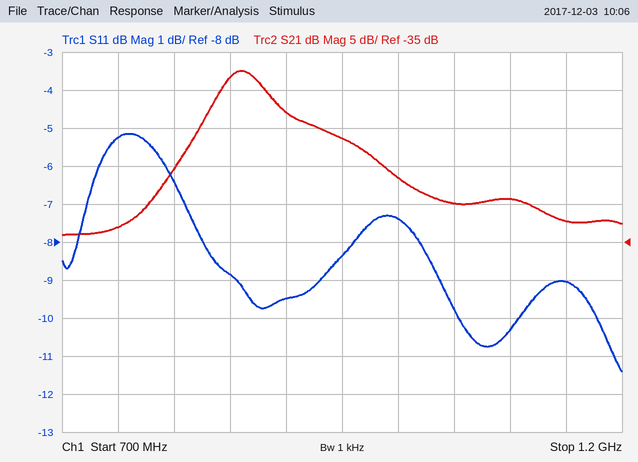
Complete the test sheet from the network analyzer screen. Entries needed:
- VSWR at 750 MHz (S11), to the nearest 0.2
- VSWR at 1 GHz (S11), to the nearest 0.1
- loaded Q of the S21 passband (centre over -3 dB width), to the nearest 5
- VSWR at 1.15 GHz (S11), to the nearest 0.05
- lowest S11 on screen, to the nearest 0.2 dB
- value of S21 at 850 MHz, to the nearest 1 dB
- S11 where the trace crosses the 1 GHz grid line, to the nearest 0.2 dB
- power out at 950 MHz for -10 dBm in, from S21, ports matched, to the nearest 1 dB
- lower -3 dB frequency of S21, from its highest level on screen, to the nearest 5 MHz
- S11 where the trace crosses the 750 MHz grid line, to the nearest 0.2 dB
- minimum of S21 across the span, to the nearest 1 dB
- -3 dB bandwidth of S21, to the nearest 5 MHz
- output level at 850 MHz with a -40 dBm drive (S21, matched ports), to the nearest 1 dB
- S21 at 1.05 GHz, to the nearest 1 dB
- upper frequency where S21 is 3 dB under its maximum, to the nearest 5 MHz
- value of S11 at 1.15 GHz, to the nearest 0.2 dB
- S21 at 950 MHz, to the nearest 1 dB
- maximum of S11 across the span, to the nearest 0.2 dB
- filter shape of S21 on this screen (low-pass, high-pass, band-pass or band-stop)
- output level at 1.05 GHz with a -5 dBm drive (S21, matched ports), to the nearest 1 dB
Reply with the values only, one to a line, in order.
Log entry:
3.4
2.5
20
2.10
-11.4 dB
-13 dB
-7.4 dB
-31 dBm
840 MHz
-5.2 dB
-34 dB
45 MHz
-53 dBm
-30 dB
885 MHz
-9.0 dB
-21 dB
-5.2 dB
band-pass
-35 dBm
